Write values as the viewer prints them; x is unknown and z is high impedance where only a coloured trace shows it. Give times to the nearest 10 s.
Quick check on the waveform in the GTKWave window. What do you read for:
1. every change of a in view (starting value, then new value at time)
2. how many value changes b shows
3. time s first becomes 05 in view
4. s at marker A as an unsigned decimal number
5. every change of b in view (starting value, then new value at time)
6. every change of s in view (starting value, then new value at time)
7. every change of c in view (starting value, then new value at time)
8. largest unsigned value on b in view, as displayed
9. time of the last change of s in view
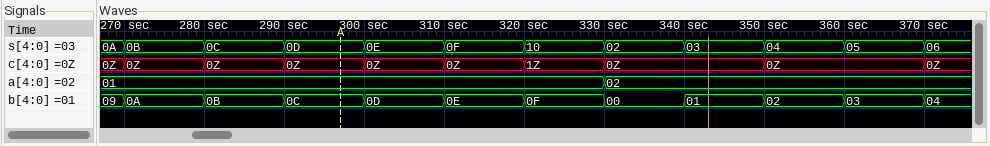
01, 02 at 330 s
11
360 s
13
09, 0A at 270 s, 0B at 280 s, 0C at 290 s, 0D at 300 s, 0E at 310 s, 0F at 320 s, 00 at 330 s, 01 at 340 s, 02 at 350 s, 03 at 360 s, 04 at 370 s
0A, 0B at 270 s, 0C at 280 s, 0D at 290 s, 0E at 300 s, 0F at 310 s, 10 at 320 s, 02 at 330 s, 03 at 340 s, 04 at 350 s, 05 at 360 s, 06 at 370 s
0Z, 0Z at 270 s, 0Z at 280 s, 0Z at 290 s, 0Z at 300 s, 0Z at 310 s, 1Z at 320 s, 0Z at 330 s, 0Z at 350 s, 0Z at 370 s
0F
370 s
